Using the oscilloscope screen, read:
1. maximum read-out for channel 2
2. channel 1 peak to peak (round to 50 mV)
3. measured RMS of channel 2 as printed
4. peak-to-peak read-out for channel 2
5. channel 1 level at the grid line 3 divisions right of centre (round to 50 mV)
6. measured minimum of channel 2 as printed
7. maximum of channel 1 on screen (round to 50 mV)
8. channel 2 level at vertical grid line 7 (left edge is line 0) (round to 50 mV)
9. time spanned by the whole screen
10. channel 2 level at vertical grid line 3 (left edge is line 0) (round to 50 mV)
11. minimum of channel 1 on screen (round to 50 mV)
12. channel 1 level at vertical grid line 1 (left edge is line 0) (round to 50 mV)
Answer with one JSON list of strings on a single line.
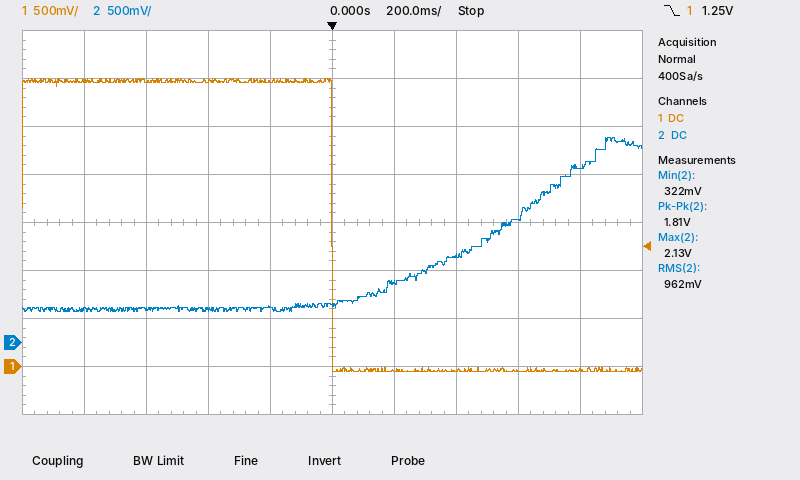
["2.13 V", "3.05 V", "962 mV", "1.81 V", "-50 mV", "322 mV", "3.00 V", "900 mV", "2 s", "350 mV", "-50 mV", "3.00 V"]
